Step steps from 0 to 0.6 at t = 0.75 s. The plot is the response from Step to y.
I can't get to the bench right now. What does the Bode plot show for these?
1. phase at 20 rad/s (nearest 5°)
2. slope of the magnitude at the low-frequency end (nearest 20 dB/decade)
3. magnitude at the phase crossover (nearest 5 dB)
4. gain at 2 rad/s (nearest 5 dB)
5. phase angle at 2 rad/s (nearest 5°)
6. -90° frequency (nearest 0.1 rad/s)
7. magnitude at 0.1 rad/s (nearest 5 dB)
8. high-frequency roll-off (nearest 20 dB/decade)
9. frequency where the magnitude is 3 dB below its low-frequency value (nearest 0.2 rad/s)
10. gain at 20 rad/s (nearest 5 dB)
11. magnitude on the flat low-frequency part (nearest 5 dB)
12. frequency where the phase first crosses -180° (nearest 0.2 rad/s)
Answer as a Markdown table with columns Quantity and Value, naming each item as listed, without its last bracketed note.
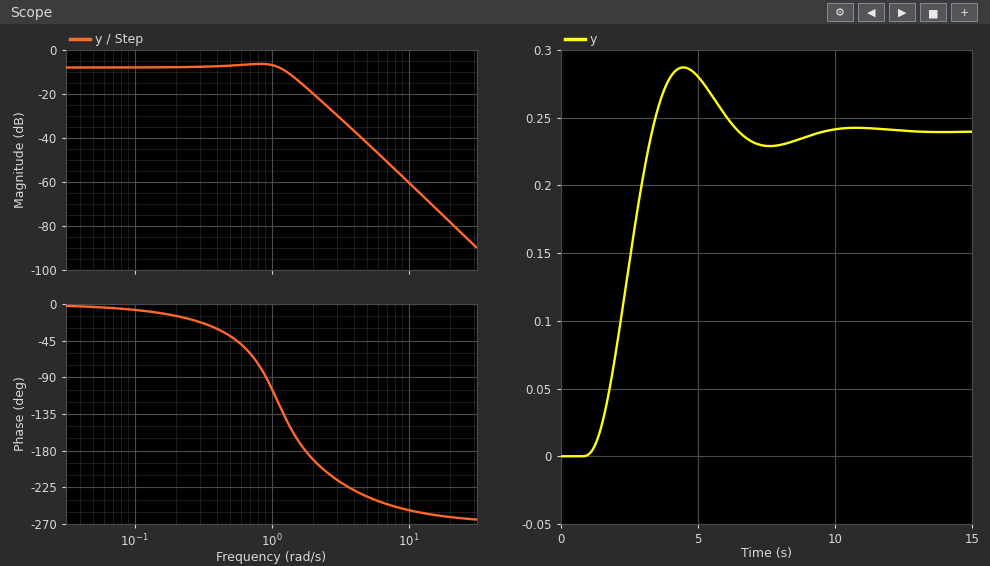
| Quantity | Value |
|---|---|
| phase at 20 rad/s | -260° |
| slope of the magnitude at the low-frequency end | 0 dB/decade |
| magnitude at the phase crossover | -15 dB |
| gain at 2 rad/s | -20 dB |
| phase angle at 2 rad/s | -190° |
| -90° frequency | 0.9 rad/s |
| magnitude at 0.1 rad/s | -10 dB |
| high-frequency roll-off | -60 dB/decade |
| frequency where the magnitude is 3 dB below its low-frequency value | 1.4 rad/s |
| gain at 20 rad/s | -80 dB |
| magnitude on the flat low-frequency part | -10 dB |
| frequency where the phase first crosses -180° | 1.8 rad/s |
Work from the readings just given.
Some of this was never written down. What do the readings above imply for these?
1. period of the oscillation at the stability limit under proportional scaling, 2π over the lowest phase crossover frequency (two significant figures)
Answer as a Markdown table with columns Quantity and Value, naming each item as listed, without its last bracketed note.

| Quantity | Value |
|---|---|
| period of the oscillation at the stability limit under proportional scaling, 2π over the lowest phase crossover frequency | 3.5 s |
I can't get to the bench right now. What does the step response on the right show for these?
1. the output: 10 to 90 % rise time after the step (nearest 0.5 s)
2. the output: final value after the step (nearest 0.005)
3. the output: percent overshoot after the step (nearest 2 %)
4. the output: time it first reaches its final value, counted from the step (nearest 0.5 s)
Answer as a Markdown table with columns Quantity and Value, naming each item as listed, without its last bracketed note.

| Quantity | Value |
|---|---|
| the output: 10 to 90 % rise time after the step | 1.5 s |
| the output: final value after the step | 0.240 |
| the output: percent overshoot after the step | 20 % |
| the output: time it first reaches its final value, counted from the step | 2.5 s |
